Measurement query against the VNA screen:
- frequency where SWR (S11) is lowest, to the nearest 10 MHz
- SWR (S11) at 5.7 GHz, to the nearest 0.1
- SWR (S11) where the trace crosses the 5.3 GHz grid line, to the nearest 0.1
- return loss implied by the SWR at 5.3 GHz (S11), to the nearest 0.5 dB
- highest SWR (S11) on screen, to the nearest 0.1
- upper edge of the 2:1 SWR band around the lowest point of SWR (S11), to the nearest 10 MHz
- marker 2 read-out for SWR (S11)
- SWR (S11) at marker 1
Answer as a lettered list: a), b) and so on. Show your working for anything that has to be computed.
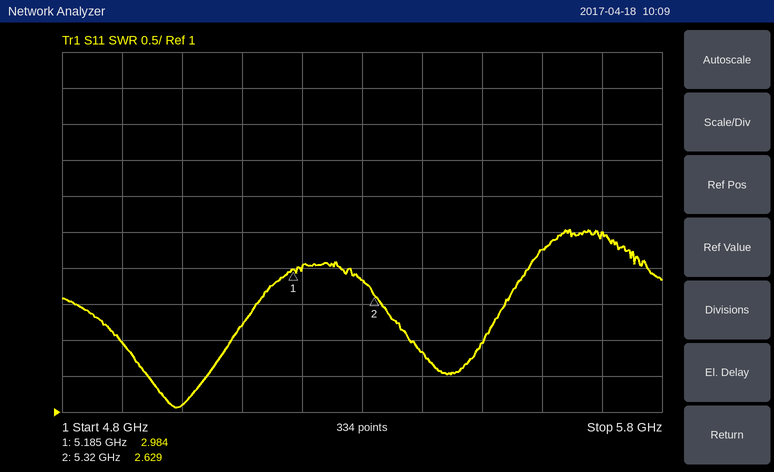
a) 4.99 GHz
b) 3.5
c) 2.8
d) −20 log10((2.8 − 1)/(2.8 + 1)) ≈ 6.5 dB
e) 3.5
f) 5.08 GHz
g) 2.629
h) 2.984
